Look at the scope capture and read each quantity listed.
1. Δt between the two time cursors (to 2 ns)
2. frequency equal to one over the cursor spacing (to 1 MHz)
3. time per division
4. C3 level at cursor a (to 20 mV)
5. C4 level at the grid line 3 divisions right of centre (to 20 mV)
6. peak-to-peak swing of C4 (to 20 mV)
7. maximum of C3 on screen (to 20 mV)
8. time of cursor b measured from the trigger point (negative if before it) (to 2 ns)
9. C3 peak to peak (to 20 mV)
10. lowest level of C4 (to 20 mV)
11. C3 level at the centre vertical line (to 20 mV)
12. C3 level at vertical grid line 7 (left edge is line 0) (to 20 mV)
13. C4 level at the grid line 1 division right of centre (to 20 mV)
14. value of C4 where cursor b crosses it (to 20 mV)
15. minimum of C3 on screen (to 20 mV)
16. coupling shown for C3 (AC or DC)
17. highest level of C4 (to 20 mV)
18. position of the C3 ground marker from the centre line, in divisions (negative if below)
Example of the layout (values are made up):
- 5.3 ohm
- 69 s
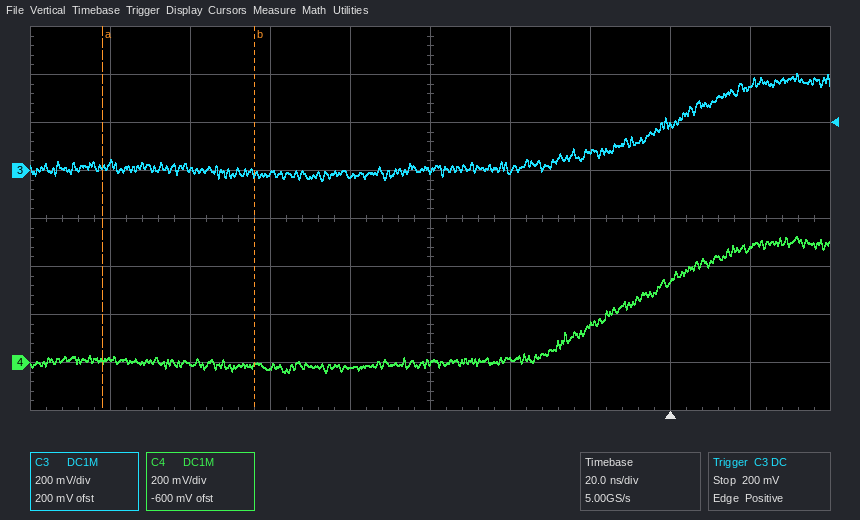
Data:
- 38 ns
- 26 MHz
- 20 ns
- 20 mV
- 340 mV
- 560 mV
- 400 mV
- -104 ns
- 440 mV
- -40 mV
- 0 mV
- 80 mV
- 20 mV
- -20 mV
- -40 mV
- DC
- 520 mV
- +1.0 div
